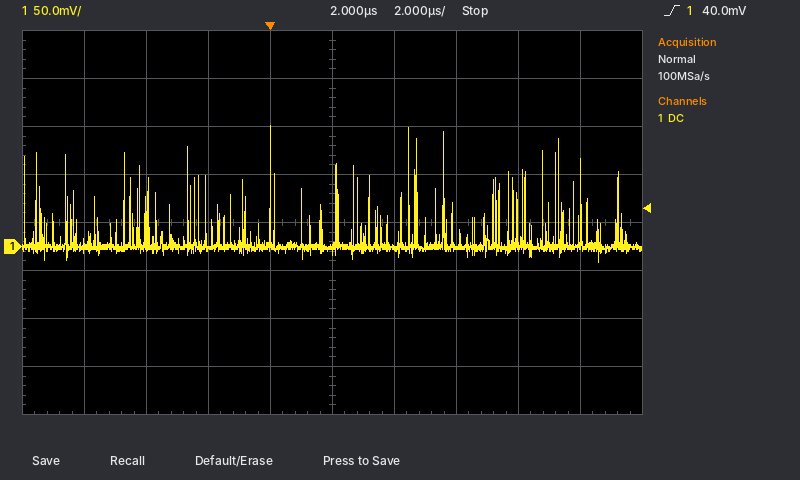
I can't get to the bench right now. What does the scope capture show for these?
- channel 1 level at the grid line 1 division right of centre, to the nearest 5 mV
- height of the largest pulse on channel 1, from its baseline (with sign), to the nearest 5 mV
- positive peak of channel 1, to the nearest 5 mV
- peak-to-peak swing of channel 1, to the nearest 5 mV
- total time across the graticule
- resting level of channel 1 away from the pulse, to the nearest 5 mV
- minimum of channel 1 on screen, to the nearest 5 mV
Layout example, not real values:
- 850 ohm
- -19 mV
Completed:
- 0 mV
- +125 mV
- 125 mV
- 140 mV
- 20 µs
- 0 mV
- -15 mV
